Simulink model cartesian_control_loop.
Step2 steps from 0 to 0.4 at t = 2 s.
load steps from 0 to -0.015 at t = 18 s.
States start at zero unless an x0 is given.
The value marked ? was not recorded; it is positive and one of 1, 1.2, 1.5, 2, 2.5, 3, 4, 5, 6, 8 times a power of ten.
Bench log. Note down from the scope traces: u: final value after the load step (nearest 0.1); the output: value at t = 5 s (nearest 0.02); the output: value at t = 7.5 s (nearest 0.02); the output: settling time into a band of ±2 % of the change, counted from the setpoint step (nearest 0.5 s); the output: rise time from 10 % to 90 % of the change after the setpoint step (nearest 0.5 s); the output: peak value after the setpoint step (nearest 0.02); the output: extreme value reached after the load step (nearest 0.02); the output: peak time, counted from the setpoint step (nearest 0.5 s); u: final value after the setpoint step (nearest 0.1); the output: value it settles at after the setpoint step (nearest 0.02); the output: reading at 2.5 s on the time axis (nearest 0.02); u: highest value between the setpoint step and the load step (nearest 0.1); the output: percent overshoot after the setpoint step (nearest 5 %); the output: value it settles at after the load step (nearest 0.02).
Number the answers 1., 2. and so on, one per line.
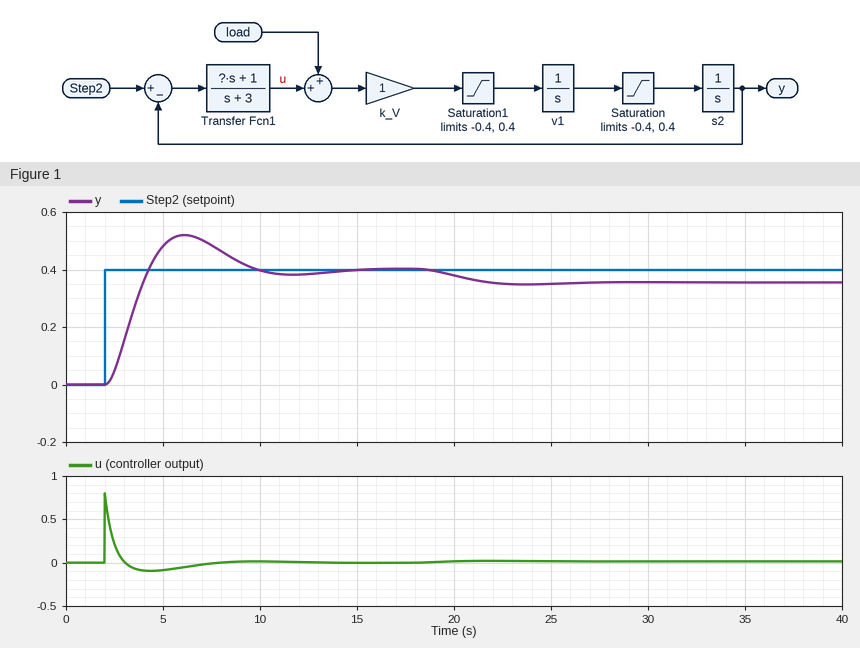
1. 0.0
2. 0.48
3. 0.48
4. 12.0 s
5. 1.5 s
6. 0.52
7. 0.34
8. 4.0 s
9. 0.0
10. 0.40
11. 0.04
12. 0.8
13. 30 %
14. 0.36
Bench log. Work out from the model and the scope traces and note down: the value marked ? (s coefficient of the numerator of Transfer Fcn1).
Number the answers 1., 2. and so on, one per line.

1. 2
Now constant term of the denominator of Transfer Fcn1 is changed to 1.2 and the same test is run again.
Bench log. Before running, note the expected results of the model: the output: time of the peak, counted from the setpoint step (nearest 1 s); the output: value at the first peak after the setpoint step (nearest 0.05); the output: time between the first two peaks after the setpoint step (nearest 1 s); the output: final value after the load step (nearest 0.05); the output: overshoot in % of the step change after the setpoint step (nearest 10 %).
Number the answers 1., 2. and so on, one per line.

1. 3 s
2. 0.60
3. 5 s
4. 0.40
5. 50 %
